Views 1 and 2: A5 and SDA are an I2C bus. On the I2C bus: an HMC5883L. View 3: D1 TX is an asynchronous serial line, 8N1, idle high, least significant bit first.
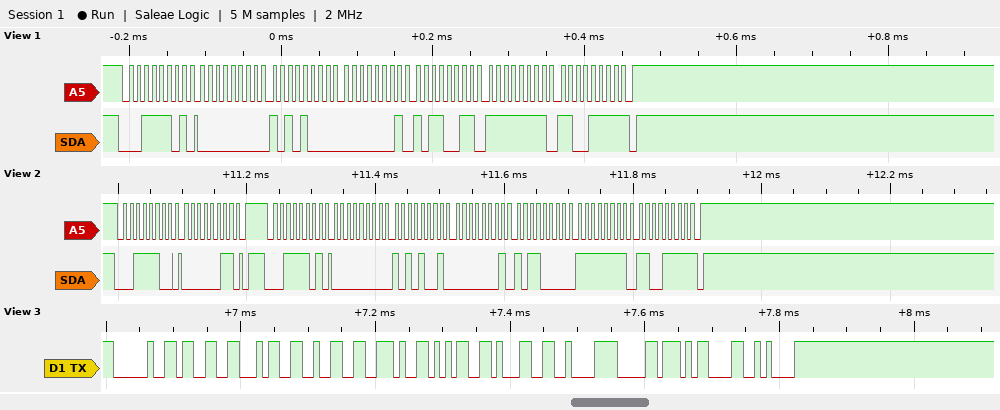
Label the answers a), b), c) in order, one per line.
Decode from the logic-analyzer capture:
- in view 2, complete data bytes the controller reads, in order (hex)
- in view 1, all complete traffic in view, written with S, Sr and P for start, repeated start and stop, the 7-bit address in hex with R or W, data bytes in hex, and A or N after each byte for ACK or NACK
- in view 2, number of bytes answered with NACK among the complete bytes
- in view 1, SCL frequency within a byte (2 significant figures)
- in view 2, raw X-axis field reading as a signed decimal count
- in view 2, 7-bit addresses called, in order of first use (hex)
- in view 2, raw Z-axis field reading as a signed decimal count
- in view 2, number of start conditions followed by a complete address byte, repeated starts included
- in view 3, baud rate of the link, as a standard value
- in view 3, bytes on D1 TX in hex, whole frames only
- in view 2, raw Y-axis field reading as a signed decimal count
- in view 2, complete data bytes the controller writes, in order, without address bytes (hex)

a) 00 A9 01 B0 FF CF
b) S 1ER A 00 A A8 A 01 A B3 A FF A CF N P
c) 1
d) 100 kHz
e) 169
f) 0x1E
g) 432
h) 2
i) 115200 baud
j) 20 33 34 32 2E 35 31 C2 B0 0D 0A
k) -49
l) 03
